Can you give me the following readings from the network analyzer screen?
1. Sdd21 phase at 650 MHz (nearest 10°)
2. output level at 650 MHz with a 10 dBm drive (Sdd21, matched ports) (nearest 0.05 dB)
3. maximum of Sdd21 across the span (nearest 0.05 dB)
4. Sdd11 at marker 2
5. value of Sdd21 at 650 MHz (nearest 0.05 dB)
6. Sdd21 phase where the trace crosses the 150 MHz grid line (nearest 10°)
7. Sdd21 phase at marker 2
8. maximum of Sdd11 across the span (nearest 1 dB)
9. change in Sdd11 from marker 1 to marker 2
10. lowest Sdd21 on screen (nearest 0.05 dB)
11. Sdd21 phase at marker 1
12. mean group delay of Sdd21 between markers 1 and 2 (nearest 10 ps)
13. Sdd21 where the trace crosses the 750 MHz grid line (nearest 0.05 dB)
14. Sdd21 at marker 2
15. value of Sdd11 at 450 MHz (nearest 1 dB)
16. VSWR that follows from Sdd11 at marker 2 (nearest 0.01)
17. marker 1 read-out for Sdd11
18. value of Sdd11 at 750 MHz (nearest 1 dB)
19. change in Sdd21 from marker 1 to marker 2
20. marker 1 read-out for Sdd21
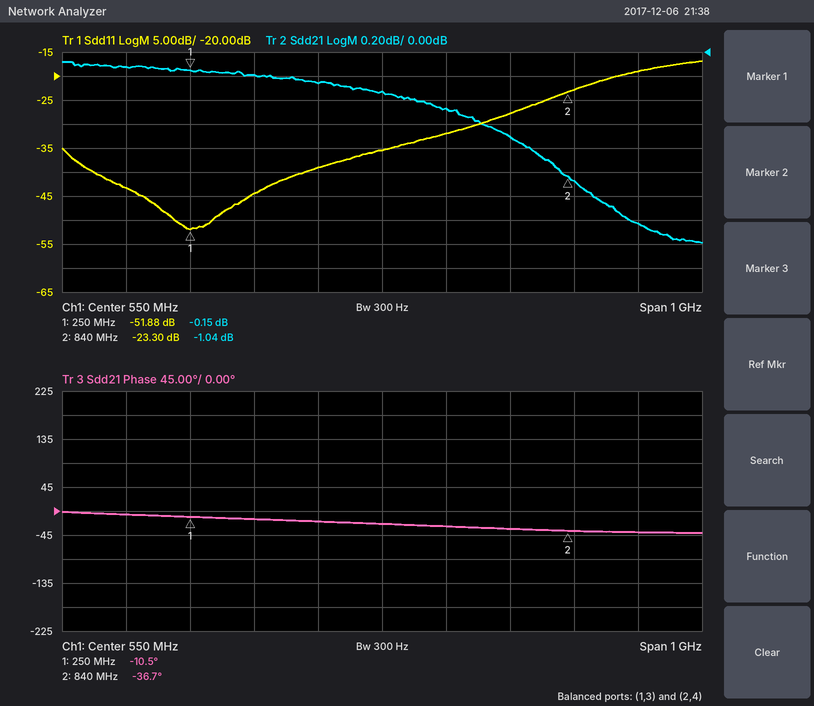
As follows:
-30°
9.55 dBm
-0.10 dB
-23.30 dB
-0.45 dB
-10°
-36.7°
-17 dB
28.58 dB
-1.60 dB
-10.5°
120 ps
-0.70 dB
-1.04 dB
-39 dB
1.15
-51.88 dB
-28 dB
-0.89 dB
-0.15 dB
